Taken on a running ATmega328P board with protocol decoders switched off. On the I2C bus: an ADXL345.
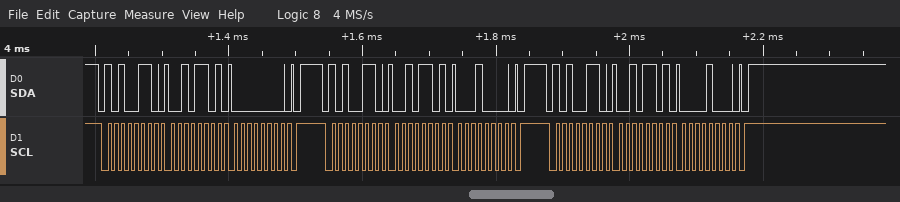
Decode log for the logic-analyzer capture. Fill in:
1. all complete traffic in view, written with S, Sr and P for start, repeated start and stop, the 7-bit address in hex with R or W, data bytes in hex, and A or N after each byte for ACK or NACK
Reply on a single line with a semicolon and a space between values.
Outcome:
S 53W A 2D A 00 A P S 53W A 2D A 10 A P S 53W A 2D A 08 A P
